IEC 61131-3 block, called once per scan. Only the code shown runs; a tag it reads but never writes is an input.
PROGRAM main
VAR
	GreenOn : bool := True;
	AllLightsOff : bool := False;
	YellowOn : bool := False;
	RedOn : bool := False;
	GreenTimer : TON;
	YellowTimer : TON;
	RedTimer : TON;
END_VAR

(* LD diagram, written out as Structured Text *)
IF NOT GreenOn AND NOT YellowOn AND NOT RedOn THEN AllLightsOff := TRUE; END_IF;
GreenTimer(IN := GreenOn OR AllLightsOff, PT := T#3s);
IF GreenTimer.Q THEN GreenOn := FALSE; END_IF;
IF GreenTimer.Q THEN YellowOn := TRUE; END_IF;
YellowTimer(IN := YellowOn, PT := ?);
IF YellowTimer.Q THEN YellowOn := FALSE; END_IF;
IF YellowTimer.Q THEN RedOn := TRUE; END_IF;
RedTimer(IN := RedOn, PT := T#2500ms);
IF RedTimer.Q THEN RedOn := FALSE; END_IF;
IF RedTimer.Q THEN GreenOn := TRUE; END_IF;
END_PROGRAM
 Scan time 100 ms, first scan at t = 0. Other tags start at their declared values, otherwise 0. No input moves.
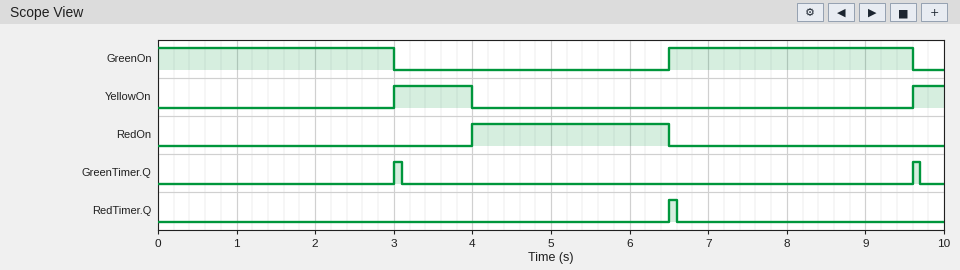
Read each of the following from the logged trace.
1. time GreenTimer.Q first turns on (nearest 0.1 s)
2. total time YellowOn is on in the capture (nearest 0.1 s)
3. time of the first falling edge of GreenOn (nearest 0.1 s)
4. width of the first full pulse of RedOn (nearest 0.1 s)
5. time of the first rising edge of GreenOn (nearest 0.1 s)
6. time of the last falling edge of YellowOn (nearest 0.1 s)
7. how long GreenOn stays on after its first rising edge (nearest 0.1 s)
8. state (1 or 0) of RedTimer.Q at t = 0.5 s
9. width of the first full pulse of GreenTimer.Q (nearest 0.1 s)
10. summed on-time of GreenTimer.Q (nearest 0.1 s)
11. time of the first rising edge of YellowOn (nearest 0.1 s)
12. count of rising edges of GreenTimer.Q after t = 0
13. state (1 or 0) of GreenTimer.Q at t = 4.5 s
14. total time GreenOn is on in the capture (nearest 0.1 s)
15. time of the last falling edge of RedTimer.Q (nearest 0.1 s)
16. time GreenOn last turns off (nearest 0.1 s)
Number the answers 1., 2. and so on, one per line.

1. 3.0 s
2. 1.4 s
3. 3.0 s
4. 2.5 s
5. 6.5 s
6. 4.0 s
7. 3.1 s
8. 0
9. 0.1 s
10. 0.2 s
11. 3.0 s
12. 2
13. 0
14. 6.1 s
15. 6.6 s
16. 9.6 s
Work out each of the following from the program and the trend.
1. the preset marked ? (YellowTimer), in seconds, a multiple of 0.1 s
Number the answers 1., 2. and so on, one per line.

1. 1.0 s
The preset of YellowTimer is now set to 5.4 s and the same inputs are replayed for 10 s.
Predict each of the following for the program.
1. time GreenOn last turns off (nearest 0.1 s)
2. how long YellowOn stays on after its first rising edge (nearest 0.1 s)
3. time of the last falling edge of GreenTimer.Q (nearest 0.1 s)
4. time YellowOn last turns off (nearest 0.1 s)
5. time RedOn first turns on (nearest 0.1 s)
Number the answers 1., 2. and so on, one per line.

1. 3.0 s
2. 5.4 s
3. 3.1 s
4. 8.4 s
5. 8.4 s
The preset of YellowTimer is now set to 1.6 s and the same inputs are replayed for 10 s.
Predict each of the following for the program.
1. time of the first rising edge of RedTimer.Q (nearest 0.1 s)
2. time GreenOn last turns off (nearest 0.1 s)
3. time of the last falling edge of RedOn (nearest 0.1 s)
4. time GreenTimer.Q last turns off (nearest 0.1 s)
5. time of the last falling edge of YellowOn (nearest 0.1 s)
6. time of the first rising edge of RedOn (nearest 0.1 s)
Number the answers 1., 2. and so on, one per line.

1. 7.1 s
2. 3.0 s
3. 7.1 s
4. 3.1 s
5. 4.6 s
6. 4.6 s
